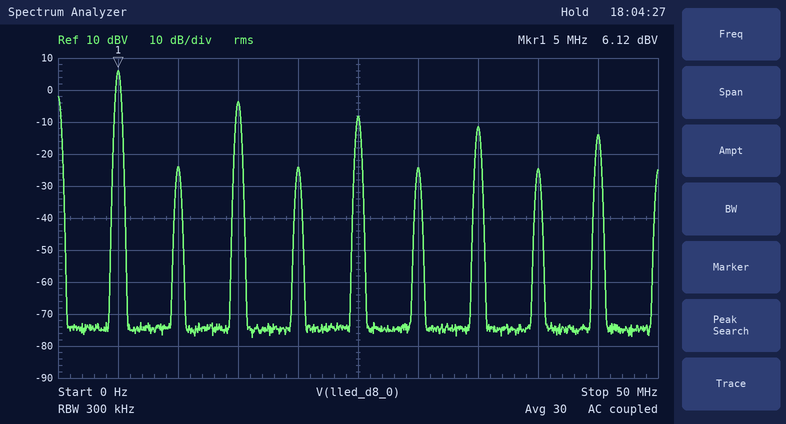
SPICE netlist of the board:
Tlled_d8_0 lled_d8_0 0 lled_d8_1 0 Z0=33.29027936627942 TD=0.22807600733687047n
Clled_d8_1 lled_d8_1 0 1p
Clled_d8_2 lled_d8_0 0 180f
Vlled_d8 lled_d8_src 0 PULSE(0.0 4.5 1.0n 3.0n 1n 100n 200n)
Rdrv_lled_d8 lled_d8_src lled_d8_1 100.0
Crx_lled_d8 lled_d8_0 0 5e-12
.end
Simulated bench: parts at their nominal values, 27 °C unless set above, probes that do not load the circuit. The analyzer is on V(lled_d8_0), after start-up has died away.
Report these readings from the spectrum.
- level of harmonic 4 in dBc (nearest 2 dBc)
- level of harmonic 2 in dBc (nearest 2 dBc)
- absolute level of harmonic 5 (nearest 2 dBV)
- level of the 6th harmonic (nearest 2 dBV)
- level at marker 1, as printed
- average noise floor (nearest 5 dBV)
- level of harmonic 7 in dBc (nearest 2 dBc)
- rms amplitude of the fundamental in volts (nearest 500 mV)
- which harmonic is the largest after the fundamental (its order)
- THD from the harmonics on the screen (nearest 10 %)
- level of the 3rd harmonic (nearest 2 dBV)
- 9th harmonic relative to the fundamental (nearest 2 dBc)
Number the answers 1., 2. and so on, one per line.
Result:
1. -30 dBc
2. -30 dBc
3. -8 dBV
4. -24 dBV
5. 6.12 dBV
6. -75 dBV
7. -18 dBc
8. 2.0 V
9. 3
10. 40 %
11. -4 dBV
12. -20 dBc
